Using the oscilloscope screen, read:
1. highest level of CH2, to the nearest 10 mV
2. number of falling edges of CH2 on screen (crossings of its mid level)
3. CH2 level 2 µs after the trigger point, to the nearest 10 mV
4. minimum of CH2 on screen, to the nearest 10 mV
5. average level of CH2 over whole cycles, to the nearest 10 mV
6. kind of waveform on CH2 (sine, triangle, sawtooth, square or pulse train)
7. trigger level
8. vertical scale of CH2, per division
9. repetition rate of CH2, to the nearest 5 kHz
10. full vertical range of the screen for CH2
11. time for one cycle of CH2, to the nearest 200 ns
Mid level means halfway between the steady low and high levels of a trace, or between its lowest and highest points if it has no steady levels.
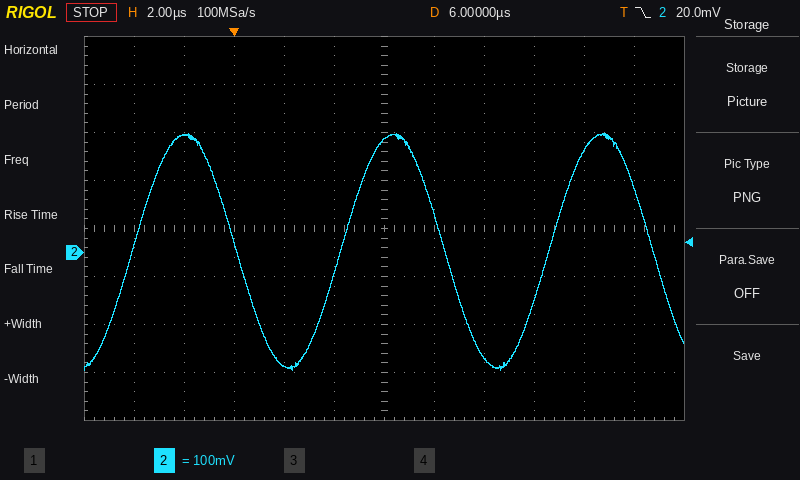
250 mV
3
-240 mV
-250 mV
0 mV
sine
20.0 mV
100 mV
120 kHz
800 mV
8.4 µs
